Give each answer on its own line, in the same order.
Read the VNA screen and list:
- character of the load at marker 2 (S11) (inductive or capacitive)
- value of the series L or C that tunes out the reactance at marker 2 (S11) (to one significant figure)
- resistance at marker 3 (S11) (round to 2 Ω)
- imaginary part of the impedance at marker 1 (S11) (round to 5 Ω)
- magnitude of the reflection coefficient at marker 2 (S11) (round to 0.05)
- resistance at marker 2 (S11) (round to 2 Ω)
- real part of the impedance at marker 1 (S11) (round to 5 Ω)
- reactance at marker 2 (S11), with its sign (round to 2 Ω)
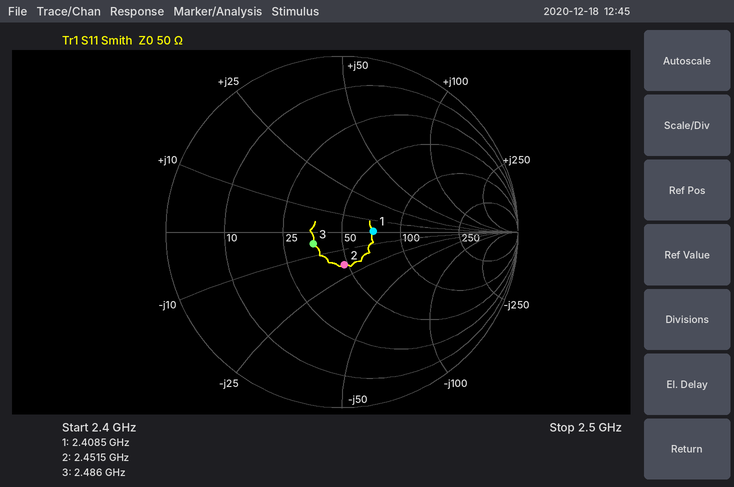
capacitive
1 nH
36 Ω
0 Ω
0.20
48 Ω
70 Ω
-18 Ω
